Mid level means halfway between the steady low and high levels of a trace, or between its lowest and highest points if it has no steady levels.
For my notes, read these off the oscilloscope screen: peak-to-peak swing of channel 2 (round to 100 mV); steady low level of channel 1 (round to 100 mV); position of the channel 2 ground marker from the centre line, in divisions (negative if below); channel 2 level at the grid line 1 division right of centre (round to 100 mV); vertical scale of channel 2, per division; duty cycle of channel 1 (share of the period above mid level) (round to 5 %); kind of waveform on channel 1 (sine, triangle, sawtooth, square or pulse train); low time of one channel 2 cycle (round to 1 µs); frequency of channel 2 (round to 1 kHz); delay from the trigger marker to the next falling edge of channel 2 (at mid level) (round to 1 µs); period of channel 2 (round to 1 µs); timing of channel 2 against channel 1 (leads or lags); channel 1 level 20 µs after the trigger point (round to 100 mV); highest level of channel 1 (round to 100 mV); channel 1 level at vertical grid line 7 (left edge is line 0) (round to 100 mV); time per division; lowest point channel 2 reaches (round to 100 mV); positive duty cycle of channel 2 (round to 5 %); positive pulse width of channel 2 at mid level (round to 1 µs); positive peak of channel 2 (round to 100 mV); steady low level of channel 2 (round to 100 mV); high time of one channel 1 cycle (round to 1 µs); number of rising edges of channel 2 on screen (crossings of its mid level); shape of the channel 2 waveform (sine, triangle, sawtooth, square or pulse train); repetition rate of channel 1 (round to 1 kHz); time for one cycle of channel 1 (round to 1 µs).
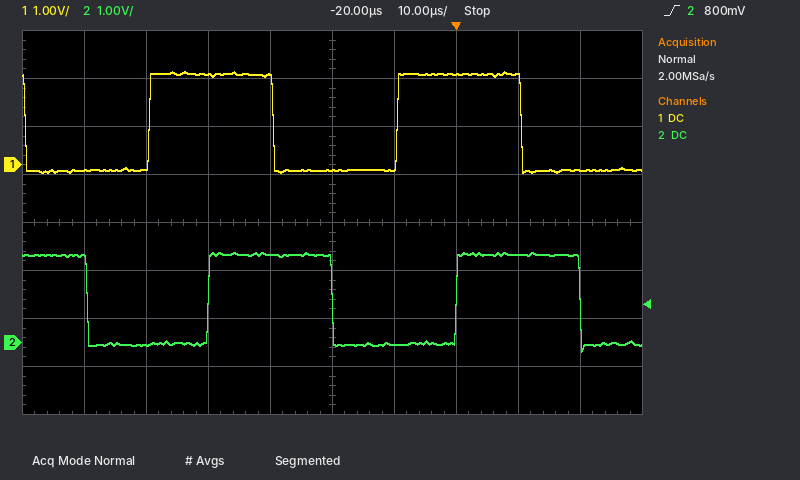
2.1 V
-100 mV
-2.5 div
0.0 V
1 V
50 %
square
20 µs
25 kHz
20 µs
40 µs
lags
-100 mV
1.9 V
1.9 V
10 µs
-200 mV
50 %
20 µs
1.9 V
0.0 V
20 µs
2
square
25 kHz
40 µs
